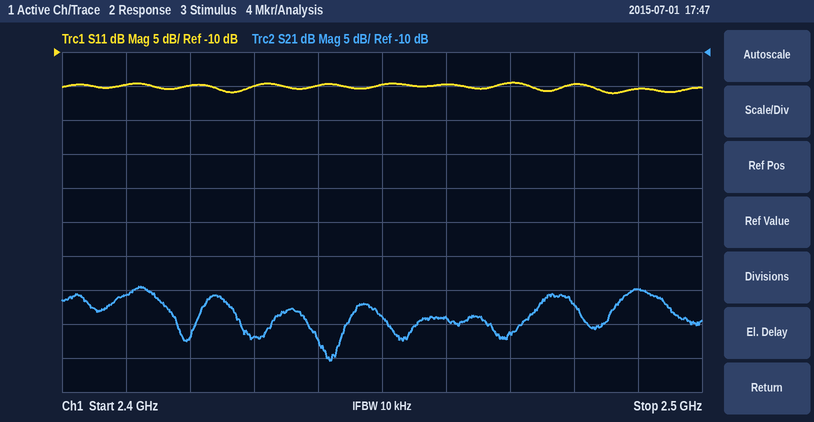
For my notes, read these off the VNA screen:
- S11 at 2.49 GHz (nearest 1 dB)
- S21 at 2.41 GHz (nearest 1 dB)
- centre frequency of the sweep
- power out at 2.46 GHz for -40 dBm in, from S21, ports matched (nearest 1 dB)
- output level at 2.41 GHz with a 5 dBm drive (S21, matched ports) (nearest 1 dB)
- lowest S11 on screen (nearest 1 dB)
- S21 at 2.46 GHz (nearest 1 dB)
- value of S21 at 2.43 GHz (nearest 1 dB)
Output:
-15 dB
-46 dB
2.45 GHz
-89 dBm
-41 dBm
-16 dB
-49 dB
-52 dB
